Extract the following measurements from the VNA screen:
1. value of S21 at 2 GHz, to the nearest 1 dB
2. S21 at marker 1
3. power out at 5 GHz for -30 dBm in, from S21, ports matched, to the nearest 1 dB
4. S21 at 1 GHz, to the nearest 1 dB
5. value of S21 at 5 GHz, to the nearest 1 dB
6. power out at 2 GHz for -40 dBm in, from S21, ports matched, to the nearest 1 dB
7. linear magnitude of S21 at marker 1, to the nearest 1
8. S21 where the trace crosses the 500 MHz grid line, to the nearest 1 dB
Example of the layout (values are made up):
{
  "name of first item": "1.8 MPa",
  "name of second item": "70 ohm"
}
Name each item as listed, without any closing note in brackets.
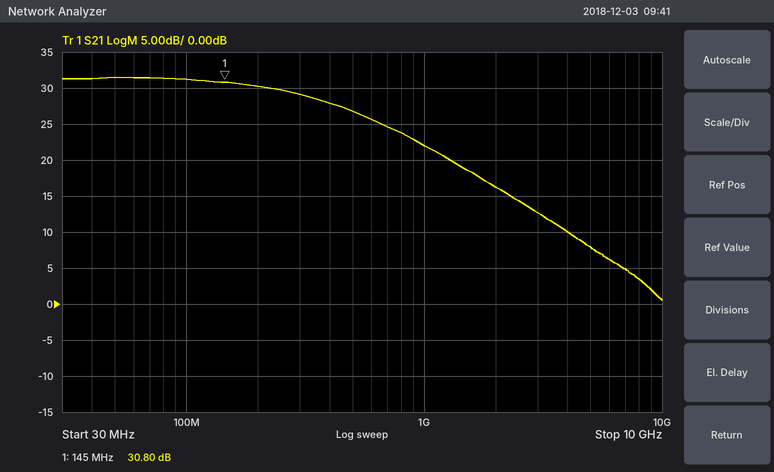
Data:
{
  "value of S21 at 2 GHz, to the nearest 1 dB": "16 dB",
  "S21 at marker 1": "30.80 dB",
  "power out at 5 GHz for -30 dBm in, from S21, ports matched, to the nearest 1 dB": "-22 dBm",
  "S21 at 1 GHz, to the nearest 1 dB": "22 dB",
  "value of S21 at 5 GHz, to the nearest 1 dB": "8 dB",
  "power out at 2 GHz for -40 dBm in, from S21, ports matched, to the nearest 1 dB": "-24 dBm",
  "linear magnitude of S21 at marker 1, to the nearest 1": "35",
  "S21 where the trace crosses the 500 MHz grid line, to the nearest 1 dB": "27 dB"
}
